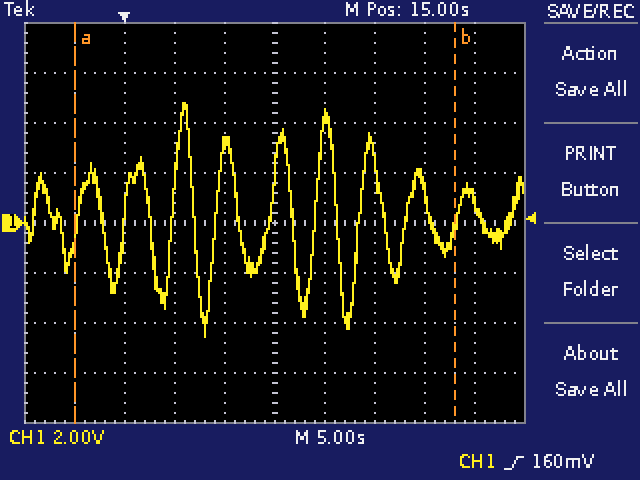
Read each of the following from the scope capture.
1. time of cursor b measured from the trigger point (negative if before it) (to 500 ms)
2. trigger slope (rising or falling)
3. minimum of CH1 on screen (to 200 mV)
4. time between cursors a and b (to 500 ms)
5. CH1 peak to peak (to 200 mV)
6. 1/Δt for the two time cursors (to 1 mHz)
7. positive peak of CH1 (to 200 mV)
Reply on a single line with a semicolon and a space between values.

+33.0 s; rising; -4.6 V; 38.0 s; 9.4 V; 26 mHz; 4.8 V
